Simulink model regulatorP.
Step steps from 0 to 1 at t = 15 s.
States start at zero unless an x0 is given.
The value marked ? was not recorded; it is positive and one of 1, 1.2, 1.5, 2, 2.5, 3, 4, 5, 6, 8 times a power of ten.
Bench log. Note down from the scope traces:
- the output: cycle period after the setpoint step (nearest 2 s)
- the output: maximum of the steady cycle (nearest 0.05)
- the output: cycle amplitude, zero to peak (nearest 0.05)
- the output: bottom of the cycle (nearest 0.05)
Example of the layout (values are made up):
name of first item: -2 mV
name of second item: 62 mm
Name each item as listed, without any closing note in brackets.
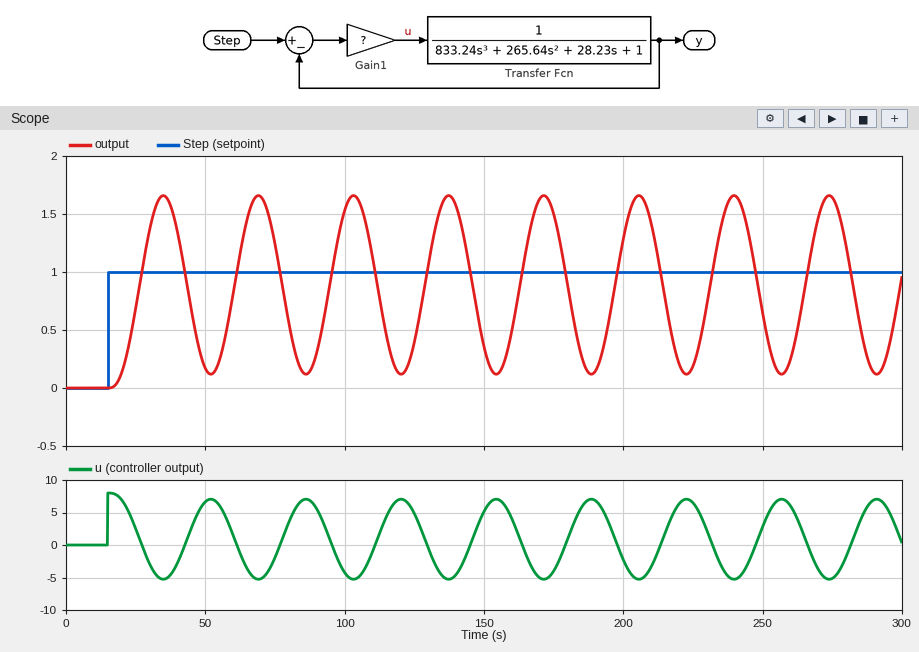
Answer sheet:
the output: cycle period after the setpoint step: 34 s
the output: maximum of the steady cycle: 1.65
the output: cycle amplitude, zero to peak: 0.75
the output: bottom of the cycle: 0.10
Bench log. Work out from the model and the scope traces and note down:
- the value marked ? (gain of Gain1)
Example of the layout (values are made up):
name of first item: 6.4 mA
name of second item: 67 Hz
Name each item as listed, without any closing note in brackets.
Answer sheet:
the value marked ?: 8
